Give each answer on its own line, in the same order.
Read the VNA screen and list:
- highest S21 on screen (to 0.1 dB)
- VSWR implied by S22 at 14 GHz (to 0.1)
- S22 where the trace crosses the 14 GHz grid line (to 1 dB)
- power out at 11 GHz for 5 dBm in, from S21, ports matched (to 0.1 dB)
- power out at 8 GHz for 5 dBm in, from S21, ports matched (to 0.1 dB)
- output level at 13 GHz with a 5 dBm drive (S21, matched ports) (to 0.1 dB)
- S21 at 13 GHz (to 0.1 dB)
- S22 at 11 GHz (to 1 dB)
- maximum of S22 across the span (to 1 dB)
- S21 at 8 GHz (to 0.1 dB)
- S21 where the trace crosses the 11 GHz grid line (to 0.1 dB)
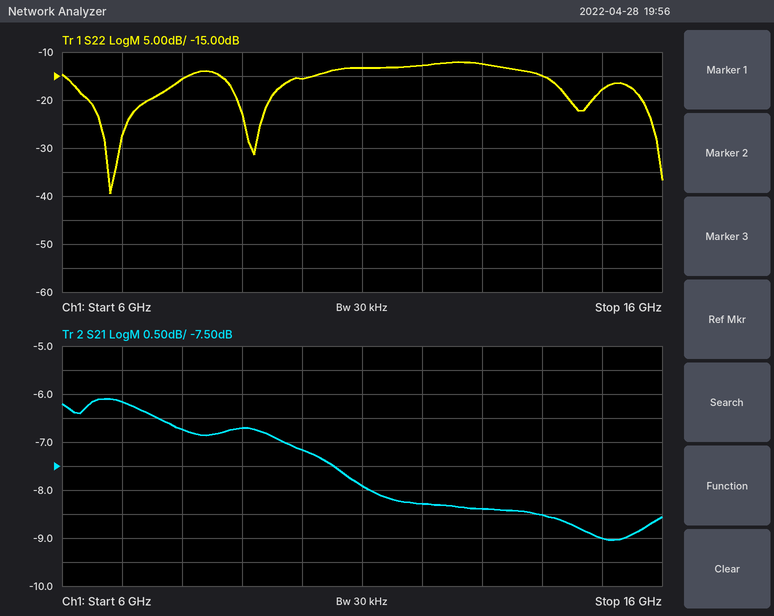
-6.1 dB
1.4
-15 dB
-2.9 dBm
-1.7 dBm
-3.4 dBm
-8.4 dB
-13 dB
-12 dB
-6.7 dB
-7.9 dB
